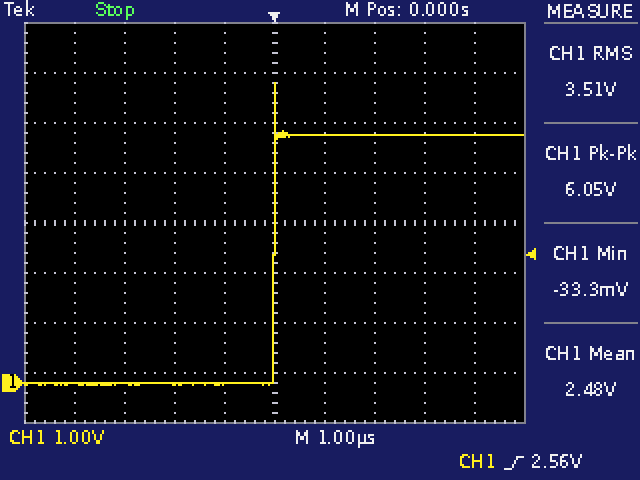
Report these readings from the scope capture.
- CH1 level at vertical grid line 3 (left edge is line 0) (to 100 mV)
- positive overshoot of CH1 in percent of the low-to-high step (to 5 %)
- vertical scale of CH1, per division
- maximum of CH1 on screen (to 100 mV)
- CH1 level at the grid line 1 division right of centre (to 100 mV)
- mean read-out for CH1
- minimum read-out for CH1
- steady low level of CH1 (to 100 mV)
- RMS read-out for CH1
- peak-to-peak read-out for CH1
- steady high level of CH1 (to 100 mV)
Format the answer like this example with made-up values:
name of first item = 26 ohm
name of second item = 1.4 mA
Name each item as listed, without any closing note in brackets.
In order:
CH1 level at vertical grid line 3 (left edge is line 0) = 0.0 V
positive overshoot of CH1 in percent of the low-to-high step = 20 %
vertical scale of CH1, per division = 1 V
maximum of CH1 on screen = 6.0 V
CH1 level at the grid line 1 division right of centre = 5.0 V
mean read-out for CH1 = 2.48 V
minimum read-out for CH1 = -33.3 mV
steady low level of CH1 = 0.0 V
RMS read-out for CH1 = 3.51 V
peak-to-peak read-out for CH1 = 6.05 V
steady high level of CH1 = 5.0 V
